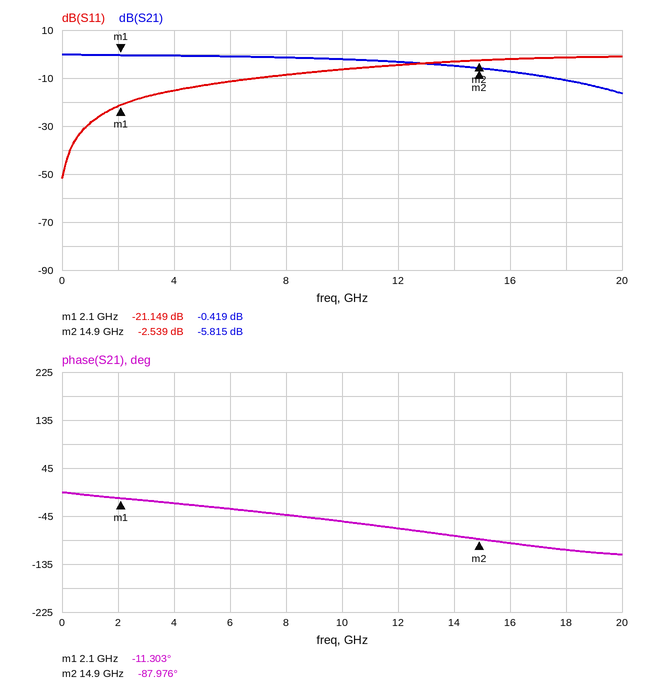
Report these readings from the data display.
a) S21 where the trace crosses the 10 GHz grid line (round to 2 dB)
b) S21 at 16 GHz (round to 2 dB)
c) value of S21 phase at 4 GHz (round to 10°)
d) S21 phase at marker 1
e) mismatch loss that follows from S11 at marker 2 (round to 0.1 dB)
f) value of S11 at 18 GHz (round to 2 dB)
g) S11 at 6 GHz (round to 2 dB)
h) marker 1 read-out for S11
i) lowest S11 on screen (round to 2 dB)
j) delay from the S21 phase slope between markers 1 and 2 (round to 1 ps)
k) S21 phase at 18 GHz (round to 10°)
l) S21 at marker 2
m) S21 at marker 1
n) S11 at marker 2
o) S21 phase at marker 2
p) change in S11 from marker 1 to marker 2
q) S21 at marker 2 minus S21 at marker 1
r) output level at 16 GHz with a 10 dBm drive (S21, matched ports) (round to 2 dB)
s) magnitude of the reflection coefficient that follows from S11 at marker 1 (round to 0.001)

-2 dB
-8 dB
-20°
-11.303°
3.5 dB
-2 dB
-12 dB
-21.149 dB
-52 dB
17 ps
-110°
-5.815 dB
-0.419 dB
-2.539 dB
-87.976°
18.610 dB
-5.396 dB
2 dBm
0.088
